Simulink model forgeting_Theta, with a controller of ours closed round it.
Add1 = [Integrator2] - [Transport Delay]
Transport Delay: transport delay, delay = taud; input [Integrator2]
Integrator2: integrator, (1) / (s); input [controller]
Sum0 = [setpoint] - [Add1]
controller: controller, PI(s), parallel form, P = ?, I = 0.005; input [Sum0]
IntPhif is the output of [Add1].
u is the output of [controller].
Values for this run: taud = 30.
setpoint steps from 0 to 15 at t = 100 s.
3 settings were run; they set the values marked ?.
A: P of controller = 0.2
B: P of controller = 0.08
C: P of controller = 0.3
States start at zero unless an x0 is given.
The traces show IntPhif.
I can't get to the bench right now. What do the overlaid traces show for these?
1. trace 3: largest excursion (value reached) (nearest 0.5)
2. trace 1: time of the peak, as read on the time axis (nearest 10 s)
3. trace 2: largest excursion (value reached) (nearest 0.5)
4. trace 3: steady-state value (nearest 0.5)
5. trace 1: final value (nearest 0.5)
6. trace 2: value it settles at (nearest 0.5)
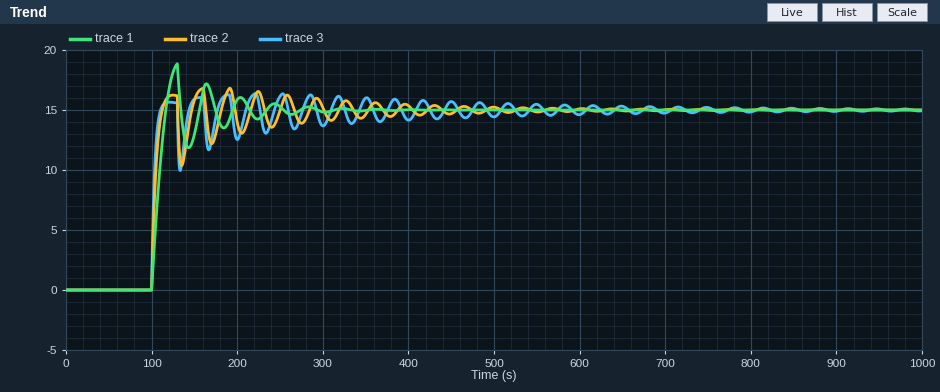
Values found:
16.5
130 s
17.0
15.0
15.0
15.0
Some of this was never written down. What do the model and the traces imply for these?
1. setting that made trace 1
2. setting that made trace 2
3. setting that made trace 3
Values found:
B
A
C
